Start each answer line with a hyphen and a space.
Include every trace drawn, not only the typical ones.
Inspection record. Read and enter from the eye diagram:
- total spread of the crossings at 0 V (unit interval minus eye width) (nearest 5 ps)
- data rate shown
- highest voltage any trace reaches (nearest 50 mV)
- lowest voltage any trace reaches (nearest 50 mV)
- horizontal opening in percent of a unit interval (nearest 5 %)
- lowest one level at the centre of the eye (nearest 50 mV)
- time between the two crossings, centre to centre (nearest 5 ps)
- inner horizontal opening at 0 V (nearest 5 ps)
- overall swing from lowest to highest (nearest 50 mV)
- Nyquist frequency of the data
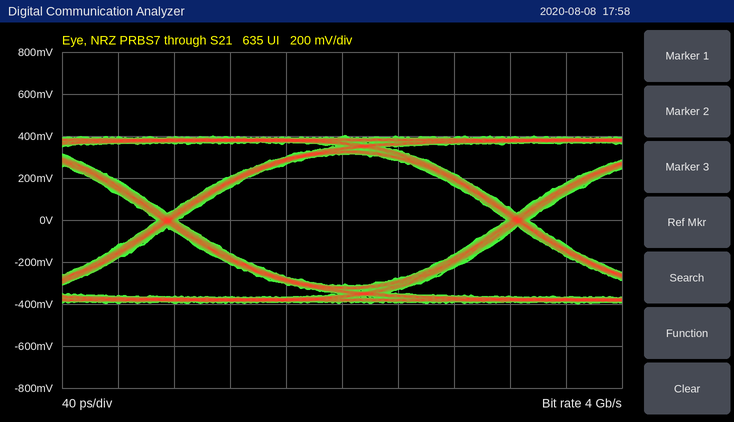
- 15 ps
- 4 Gb/s
- 400 mV
- -400 mV
- 95 %
- 300 mV
- 250 ps
- 235 ps
- 800 mV
- 2 GHz
